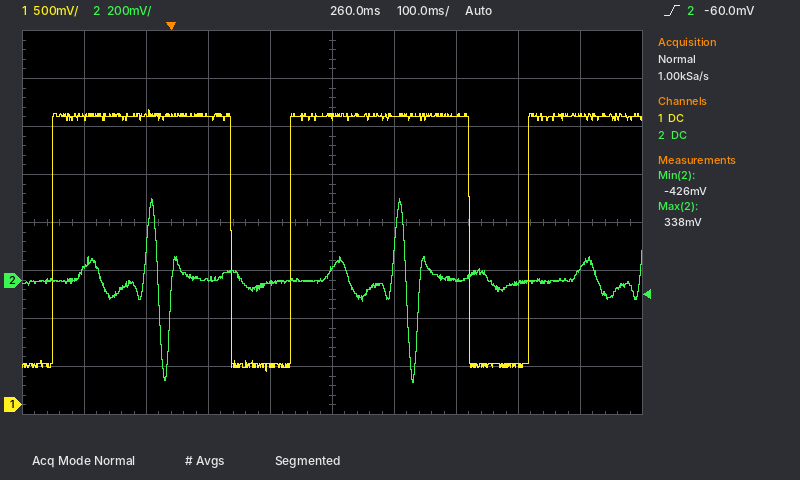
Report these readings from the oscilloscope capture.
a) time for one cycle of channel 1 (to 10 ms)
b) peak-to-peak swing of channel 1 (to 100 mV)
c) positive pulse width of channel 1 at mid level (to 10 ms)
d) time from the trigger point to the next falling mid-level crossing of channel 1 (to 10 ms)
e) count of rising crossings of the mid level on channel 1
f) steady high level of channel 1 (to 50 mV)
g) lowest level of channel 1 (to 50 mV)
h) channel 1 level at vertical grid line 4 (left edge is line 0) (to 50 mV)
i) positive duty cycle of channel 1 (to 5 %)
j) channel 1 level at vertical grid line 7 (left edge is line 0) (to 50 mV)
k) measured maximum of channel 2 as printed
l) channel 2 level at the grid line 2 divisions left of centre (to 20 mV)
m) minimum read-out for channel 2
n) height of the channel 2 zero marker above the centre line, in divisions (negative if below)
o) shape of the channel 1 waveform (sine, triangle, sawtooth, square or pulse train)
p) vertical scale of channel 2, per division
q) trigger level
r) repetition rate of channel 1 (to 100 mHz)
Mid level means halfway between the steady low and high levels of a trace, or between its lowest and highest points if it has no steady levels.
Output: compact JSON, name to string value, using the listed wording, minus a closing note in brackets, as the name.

{"time for one cycle of channel 1": "380 ms", "peak-to-peak swing of channel 1": "2.70 V", "positive pulse width of channel 1 at mid level": "290 ms", "time from the trigger point to the next falling mid-level crossing of channel 1": "100 ms", "count of rising crossings of the mid level on channel 1": "3", "steady high level of channel 1": "3.00 V", "lowest level of channel 1": "350 mV", "channel 1 level at vertical grid line 4 (left edge is line 0)": "400 mV", "positive duty cycle of channel 1": "75 %", "channel 1 level at vertical grid line 7 (left edge is line 0)": "3.00 V", "measured maximum of channel 2 as printed": "338 mV", "channel 2 level at the grid line 2 divisions left of centre": "0 mV", "minimum read-out for channel 2": "-426 mV", "height of the channel 2 zero marker above the centre line, in divisions": "-1.2 div", "shape of the channel 1 waveform": "pulse train", "vertical scale of channel 2, per division": "200 mV", "trigger level": "-60.0 mV", "repetition rate of channel 1": "2.6 Hz"}
